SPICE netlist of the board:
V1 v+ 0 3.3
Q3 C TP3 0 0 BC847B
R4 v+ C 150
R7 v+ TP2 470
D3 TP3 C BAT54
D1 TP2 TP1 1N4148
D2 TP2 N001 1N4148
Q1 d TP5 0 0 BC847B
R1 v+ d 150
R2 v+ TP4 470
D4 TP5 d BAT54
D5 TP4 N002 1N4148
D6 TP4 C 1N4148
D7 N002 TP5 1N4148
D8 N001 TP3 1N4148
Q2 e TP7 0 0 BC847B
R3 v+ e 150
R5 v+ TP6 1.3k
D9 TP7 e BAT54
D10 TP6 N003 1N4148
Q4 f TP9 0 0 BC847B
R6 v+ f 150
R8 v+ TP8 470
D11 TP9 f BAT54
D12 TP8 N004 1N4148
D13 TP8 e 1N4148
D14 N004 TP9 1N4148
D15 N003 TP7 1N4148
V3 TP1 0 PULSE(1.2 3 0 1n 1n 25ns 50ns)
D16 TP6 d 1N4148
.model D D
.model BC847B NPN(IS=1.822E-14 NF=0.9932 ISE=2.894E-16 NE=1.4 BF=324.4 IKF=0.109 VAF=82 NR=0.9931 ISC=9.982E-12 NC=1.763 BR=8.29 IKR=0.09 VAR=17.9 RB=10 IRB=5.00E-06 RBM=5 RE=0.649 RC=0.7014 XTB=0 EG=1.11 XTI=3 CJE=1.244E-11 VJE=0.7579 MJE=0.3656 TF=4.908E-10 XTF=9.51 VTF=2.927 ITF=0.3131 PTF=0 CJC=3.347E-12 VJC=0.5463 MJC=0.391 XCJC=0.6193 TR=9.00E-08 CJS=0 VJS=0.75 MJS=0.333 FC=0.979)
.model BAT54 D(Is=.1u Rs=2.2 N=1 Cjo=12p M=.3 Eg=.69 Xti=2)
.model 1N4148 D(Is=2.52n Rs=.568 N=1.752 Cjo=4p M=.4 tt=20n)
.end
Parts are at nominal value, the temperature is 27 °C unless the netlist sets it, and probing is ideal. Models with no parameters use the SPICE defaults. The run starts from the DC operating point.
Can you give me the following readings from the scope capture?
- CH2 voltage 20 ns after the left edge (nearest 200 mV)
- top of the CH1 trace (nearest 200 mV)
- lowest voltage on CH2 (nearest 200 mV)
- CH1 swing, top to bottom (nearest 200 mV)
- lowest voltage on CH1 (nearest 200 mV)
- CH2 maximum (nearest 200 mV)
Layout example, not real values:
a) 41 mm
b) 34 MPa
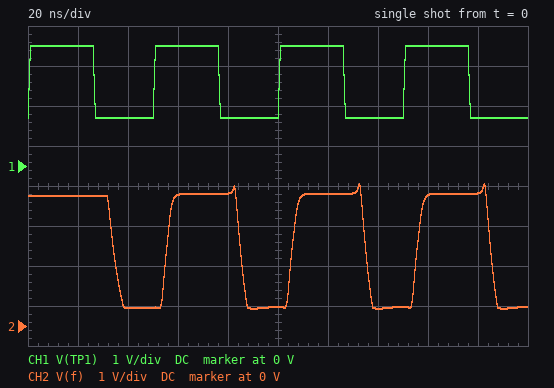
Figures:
a) 3.2 V
b) 3.0 V
c) 400 mV
d) 1.8 V
e) 1.2 V
f) 3.6 V
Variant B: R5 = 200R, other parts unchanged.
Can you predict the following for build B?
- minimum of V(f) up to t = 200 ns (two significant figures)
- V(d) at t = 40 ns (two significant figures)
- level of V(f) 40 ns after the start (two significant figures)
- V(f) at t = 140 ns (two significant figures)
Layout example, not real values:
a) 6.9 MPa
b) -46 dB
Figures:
a) 390 mV
b) 540 mV
c) 420 mV
d) 430 mV
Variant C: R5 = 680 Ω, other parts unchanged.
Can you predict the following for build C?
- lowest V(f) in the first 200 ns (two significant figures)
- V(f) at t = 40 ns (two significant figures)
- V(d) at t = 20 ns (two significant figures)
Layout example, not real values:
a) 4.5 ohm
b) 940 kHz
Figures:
a) 390 mV
b) 440 mV
c) 3.2 V
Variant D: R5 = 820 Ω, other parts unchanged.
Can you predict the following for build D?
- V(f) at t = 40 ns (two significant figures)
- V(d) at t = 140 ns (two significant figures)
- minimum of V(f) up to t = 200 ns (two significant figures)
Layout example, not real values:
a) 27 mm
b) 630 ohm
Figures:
a) 440 mV
b) 470 mV
c) 390 mV
